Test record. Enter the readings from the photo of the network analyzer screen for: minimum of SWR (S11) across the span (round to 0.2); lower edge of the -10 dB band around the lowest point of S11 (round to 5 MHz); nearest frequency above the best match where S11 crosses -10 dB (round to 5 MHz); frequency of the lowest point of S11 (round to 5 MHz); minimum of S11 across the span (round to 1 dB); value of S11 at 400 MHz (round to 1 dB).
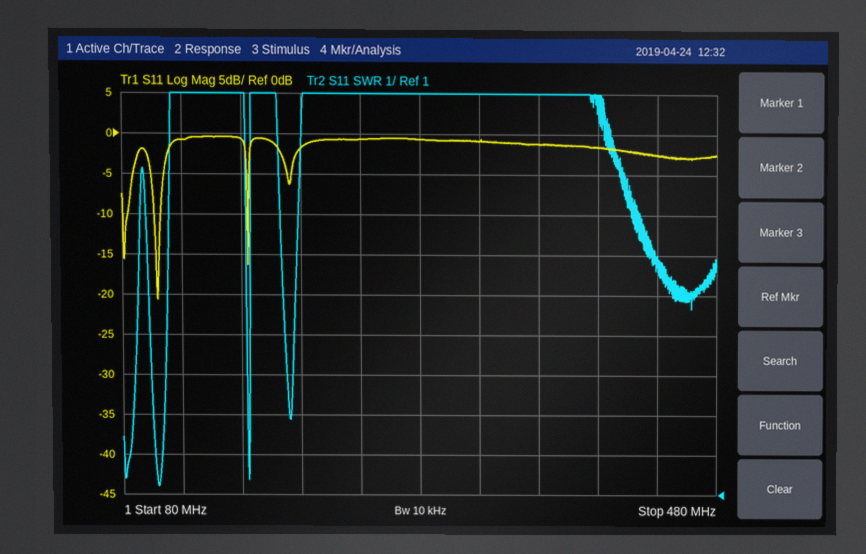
1.2
100 MHz
105 MHz
105 MHz
-21 dB
-2 dB
